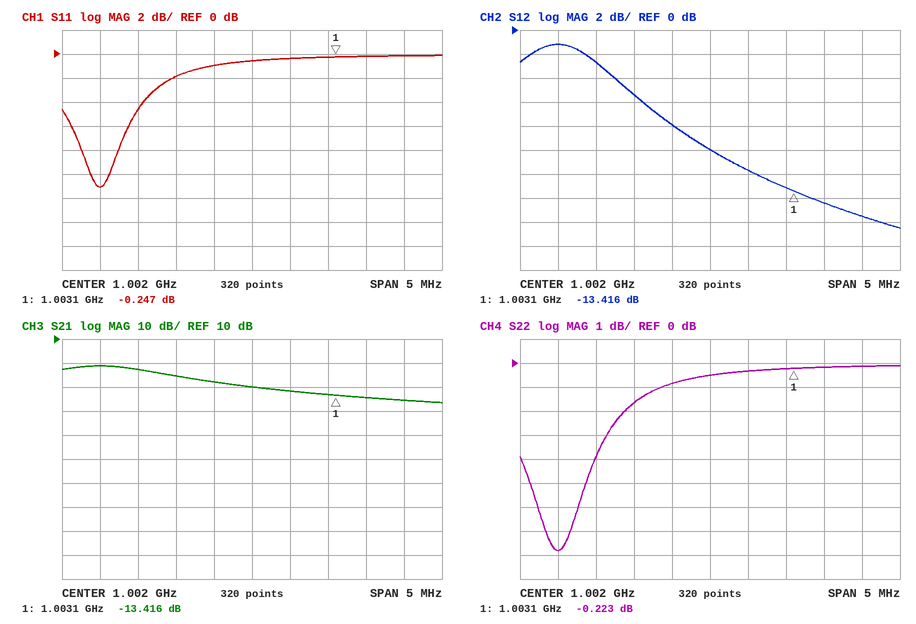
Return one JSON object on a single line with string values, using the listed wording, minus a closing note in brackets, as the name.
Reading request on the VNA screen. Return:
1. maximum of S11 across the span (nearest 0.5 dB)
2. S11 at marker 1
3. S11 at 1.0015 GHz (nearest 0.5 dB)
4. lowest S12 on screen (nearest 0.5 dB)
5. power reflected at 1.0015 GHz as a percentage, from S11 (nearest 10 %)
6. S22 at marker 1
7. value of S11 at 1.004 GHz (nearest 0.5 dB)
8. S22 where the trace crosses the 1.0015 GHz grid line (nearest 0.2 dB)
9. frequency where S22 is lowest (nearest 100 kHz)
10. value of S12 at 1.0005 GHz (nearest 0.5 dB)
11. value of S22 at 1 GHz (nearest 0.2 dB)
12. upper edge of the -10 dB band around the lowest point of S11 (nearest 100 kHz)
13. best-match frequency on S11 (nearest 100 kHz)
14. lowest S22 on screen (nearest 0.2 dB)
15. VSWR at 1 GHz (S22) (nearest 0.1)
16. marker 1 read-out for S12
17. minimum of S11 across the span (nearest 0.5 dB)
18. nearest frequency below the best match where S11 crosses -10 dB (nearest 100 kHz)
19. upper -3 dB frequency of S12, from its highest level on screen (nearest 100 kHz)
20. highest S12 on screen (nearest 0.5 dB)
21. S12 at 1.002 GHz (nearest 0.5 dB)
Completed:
{"maximum of S11 across the span": "0.0 dB", "S11 at marker 1": "-0.247 dB", "S11 at 1.0015 GHz": "-1.0 dB", "lowest S12 on screen": "-16.5 dB", "power reflected at 1.0015 GHz as a percentage, from S11": "80 %", "S22 at marker 1": "-0.223 dB", "value of S11 at 1.004 GHz": "0.0 dB", "S22 where the trace crosses the 1.0015 GHz grid line": "-0.8 dB", "frequency where S22 is lowest": "1.0000 GHz", "value of S12 at 1.0005 GHz": "-2.5 dB", "value of S22 at 1 GHz": "-7.8 dB", "upper edge of the -10 dB band around the lowest point of S11": "1.0001 GHz", "best-match frequency on S11": "1.0000 GHz", "lowest S22 on screen": "-7.8 dB", "VSWR at 1 GHz (S22)": "2.4", "marker 1 read-out for S12": "-13.416 dB", "minimum of S11 across the span": "-11.0 dB", "nearest frequency below the best match where S11 crosses -10 dB": "999.9 MHz", "upper -3 dB frequency of S12, from its highest level on screen": "1.0008 GHz", "highest S12 on screen": "-1.0 dB", "S12 at 1.002 GHz": "-10.0 dB"}
